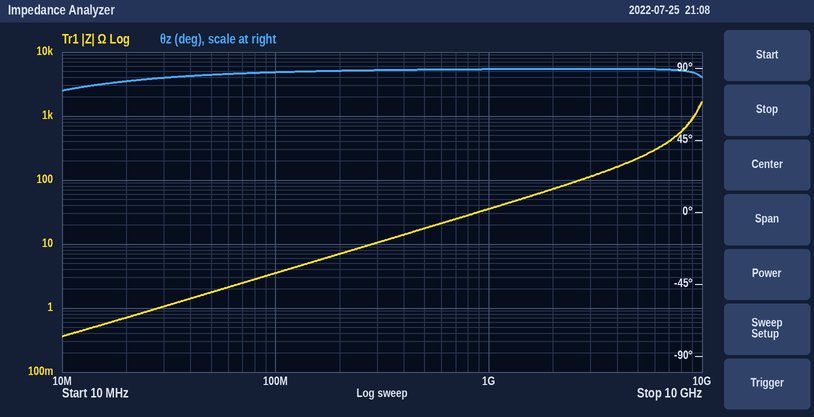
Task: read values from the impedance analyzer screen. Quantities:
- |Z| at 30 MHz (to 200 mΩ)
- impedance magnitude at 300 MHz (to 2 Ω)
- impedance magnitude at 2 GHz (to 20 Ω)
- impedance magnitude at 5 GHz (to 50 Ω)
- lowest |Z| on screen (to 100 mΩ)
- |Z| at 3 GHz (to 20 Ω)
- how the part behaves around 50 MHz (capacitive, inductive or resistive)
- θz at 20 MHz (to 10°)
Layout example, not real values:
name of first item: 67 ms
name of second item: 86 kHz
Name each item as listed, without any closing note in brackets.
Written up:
|Z| at 30 MHz: 1.0 Ω
impedance magnitude at 300 MHz: 10 Ω
impedance magnitude at 2 GHz: 80 Ω
impedance magnitude at 5 GHz: 200 Ω
lowest |Z| on screen: 400 mΩ
|Z| at 3 GHz: 120 Ω
how the part behaves around 50 MHz: inductive
θz at 20 MHz: 80°
